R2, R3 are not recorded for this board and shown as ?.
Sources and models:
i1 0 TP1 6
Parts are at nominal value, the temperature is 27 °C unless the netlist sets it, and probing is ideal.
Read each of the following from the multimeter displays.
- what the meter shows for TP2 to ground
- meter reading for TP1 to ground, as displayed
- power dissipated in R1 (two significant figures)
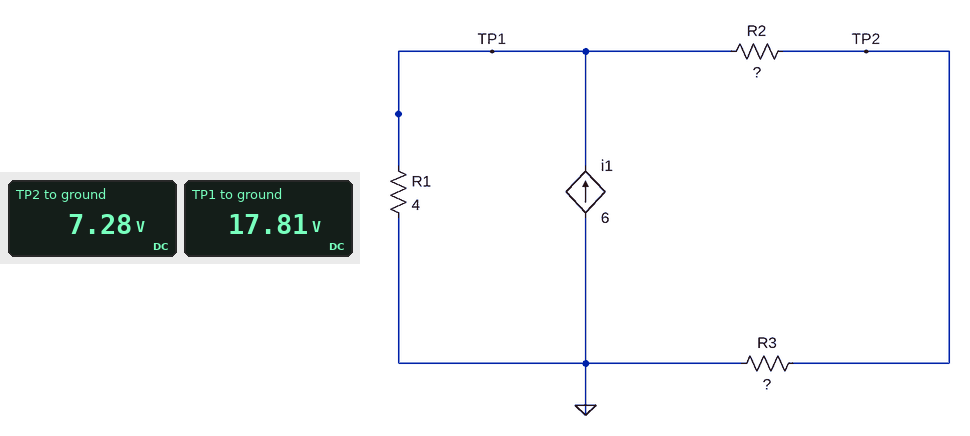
7.28 V
17.81 V
79 W
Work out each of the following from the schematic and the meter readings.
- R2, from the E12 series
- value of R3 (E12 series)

6.8 Ω
4.7 Ω
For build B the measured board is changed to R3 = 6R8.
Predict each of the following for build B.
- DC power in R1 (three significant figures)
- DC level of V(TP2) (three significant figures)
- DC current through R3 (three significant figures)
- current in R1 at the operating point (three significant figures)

86.0 W
9.27 V
1.36 A
4.64 A
